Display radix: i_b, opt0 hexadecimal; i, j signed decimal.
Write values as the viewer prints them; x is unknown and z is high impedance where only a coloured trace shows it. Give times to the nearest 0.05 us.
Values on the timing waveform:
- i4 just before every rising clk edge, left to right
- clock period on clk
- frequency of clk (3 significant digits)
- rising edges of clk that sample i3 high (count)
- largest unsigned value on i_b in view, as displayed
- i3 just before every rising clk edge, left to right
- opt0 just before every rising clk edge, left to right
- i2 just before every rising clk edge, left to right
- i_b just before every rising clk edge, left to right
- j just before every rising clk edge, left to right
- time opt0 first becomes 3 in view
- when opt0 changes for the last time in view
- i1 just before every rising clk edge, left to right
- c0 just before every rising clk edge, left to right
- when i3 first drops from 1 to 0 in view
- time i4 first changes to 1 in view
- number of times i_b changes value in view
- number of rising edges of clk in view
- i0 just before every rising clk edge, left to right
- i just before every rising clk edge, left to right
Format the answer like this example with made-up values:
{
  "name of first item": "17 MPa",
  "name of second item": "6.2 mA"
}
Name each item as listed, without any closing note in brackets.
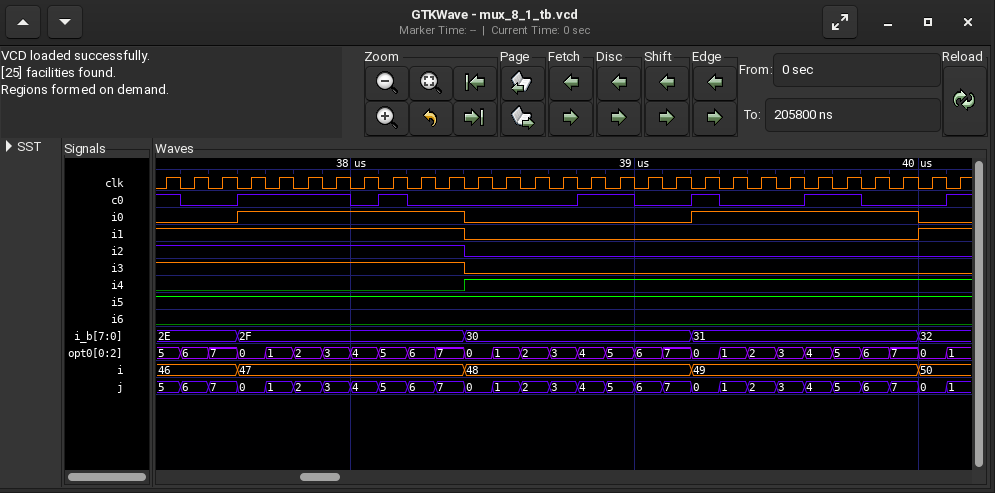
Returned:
{
  "i4 just before every rising clk edge, left to right": "0 0 0 0 0 0 0 0 0 0 0 1 1 1 1 1 1 1 1 1 1 1 1 1 1 1 1 1 1",
  "clock period on clk": "0.1 us",
  "frequency of clk": "10.0 MHz",
  "rising edges of clk that sample i3 high": "11",
  "largest unsigned value on i_b in view, as displayed": "32",
  "i3 just before every rising clk edge, left to right": "1 1 1 1 1 1 1 1 1 1 1 0 0 0 0 0 0 0 0 0 0 0 0 0 0 0 0 0 0",
  "opt0 just before every rising clk edge, left to right": "5, 6, 7, 0, 1, 2, 3, 4, 5, 6, 7, 0, 1, 2, 3, 4, 5, 6, 7, 0, 1, 2, 3, 4, 5, 6, 7, 0, 1",
  "i2 just before every rising clk edge, left to right": "1 1 1 1 1 1 1 1 1 1 1 0 0 0 0 0 0 0 0 0 0 0 0 0 0 0 0 0 0",
  "i_b just before every rising clk edge, left to right": "2E, 2E, 2E, 2F, 2F, 2F, 2F, 2F, 2F, 2F, 2F, 30, 30, 30, 30, 30, 30, 30, 30, 31, 31, 31, 31, 31, 31, 31, 31, 32, 32",
  "j just before every rising clk edge, left to right": "5, 6, 7, 0, 1, 2, 3, 4, 5, 6, 7, 0, 1, 2, 3, 4, 5, 6, 7, 0, 1, 2, 3, 4, 5, 6, 7, 0, 1",
  "time opt0 first becomes 3 in view": "37.9 us",
  "when opt0 changes for the last time in view": "40.1 us",
  "i1 just before every rising clk edge, left to right": "1 1 1 1 1 1 1 1 1 1 1 0 0 0 0 0 0 0 0 0 0 0 0 0 0 0 0 1 1",
  "c0 just before every rising clk edge, left to right": "1 0 0 1 1 1 1 0 1 0 0 0 0 0 0 1 1 0 0 1 0 0 0 1 1 0 0 0 1",
  "when i3 first drops from 1 to 0 in view": "38.4 us",
  "time i4 first changes to 1 in view": "38.4 us",
  "number of times i_b changes value in view": "4",
  "number of rising edges of clk in view": "29",
  "i0 just before every rising clk edge, left to right": "0 0 0 1 1 1 1 1 1 1 1 0 0 0 0 0 0 0 0 1 1 1 1 1 1 1 1 0 0",
  "i just before every rising clk edge, left to right": "46, 46, 46, 47, 47, 47, 47, 47, 47, 47, 47, 48, 48, 48, 48, 48, 48, 48, 48, 49, 49, 49, 49, 49, 49, 49, 49, 50, 50"
}
